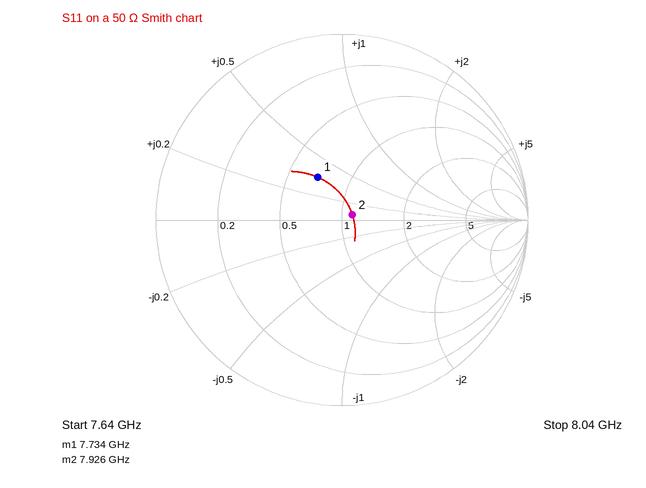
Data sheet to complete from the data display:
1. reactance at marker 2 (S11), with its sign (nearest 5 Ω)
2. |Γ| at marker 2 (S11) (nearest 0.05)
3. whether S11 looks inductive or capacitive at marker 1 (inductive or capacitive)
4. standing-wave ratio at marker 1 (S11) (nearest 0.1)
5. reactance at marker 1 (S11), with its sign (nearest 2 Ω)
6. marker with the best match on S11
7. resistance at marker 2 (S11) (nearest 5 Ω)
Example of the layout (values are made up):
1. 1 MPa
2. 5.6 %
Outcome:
1. +5 Ω
2. 0.05
3. inductive
4. 1.7
5. +18 Ω
6. marker 2
7. 55 Ω
